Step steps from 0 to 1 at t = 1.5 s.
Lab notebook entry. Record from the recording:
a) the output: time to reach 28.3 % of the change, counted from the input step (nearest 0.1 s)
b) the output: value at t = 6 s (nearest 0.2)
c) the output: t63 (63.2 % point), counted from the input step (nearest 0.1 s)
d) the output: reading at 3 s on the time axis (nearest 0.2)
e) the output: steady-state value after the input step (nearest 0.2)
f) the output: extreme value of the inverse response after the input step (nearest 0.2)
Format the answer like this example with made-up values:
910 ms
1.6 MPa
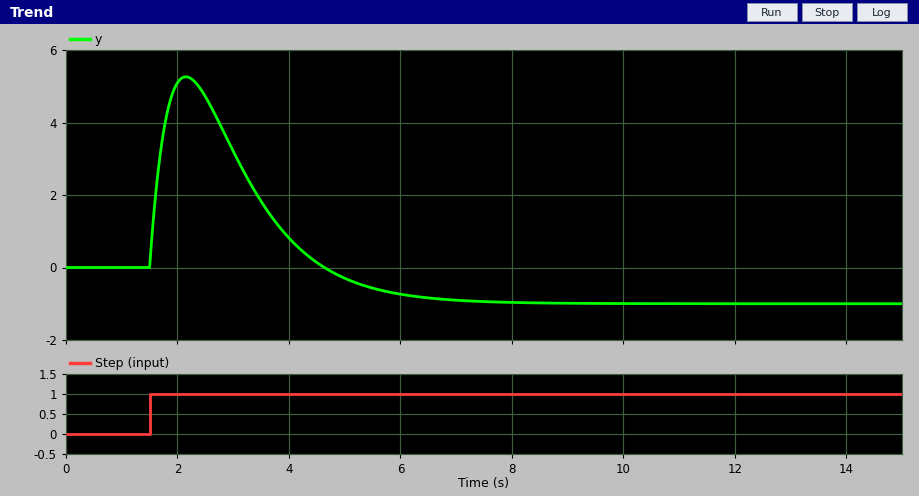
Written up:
3.5 s
-0.8
4.2 s
3.2
-1.0
5.2
